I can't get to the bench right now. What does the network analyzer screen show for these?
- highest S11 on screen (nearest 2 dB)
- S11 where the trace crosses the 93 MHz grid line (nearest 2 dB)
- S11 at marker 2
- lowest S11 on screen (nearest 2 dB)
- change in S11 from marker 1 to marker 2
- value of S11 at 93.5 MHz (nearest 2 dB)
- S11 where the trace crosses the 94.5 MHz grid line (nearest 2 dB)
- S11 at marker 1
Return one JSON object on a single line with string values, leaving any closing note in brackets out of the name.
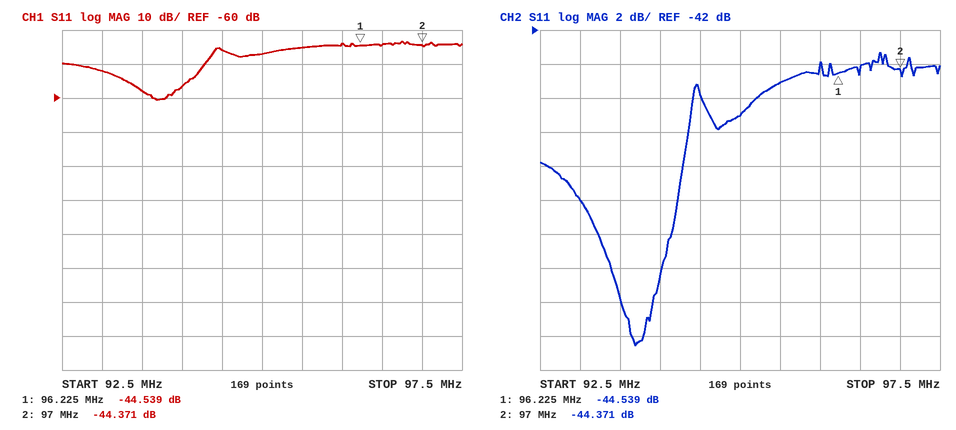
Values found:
{"highest S11 on screen": "-44 dB", "S11 where the trace crosses the 93 MHz grid line": "-52 dB", "S11 at marker 2": "-44.371 dB", "lowest S11 on screen": "-60 dB", "change in S11 from marker 1 to marker 2": "0.168 dB", "value of S11 at 93.5 MHz": "-58 dB", "S11 where the trace crosses the 94.5 MHz grid line": "-46 dB", "S11 at marker 1": "-44.539 dB"}
